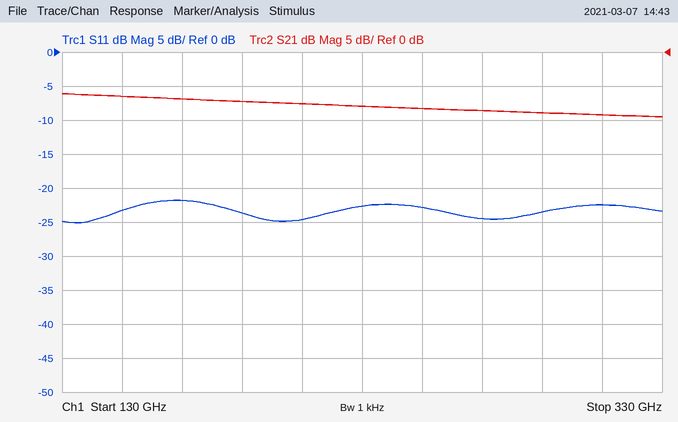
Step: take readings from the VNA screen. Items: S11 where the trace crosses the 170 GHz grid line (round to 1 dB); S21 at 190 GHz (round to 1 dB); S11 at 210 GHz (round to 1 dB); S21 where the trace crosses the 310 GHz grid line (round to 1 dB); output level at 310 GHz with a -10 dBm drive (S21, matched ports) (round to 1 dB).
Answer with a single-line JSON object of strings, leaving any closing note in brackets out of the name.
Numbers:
{"S11 where the trace crosses the 170 GHz grid line": "-22 dB", "S21 at 190 GHz": "-7 dB", "S11 at 210 GHz": "-25 dB", "S21 where the trace crosses the 310 GHz grid line": "-9 dB", "output level at 310 GHz with a -10 dBm drive (S21, matched ports)": "-19 dBm"}
